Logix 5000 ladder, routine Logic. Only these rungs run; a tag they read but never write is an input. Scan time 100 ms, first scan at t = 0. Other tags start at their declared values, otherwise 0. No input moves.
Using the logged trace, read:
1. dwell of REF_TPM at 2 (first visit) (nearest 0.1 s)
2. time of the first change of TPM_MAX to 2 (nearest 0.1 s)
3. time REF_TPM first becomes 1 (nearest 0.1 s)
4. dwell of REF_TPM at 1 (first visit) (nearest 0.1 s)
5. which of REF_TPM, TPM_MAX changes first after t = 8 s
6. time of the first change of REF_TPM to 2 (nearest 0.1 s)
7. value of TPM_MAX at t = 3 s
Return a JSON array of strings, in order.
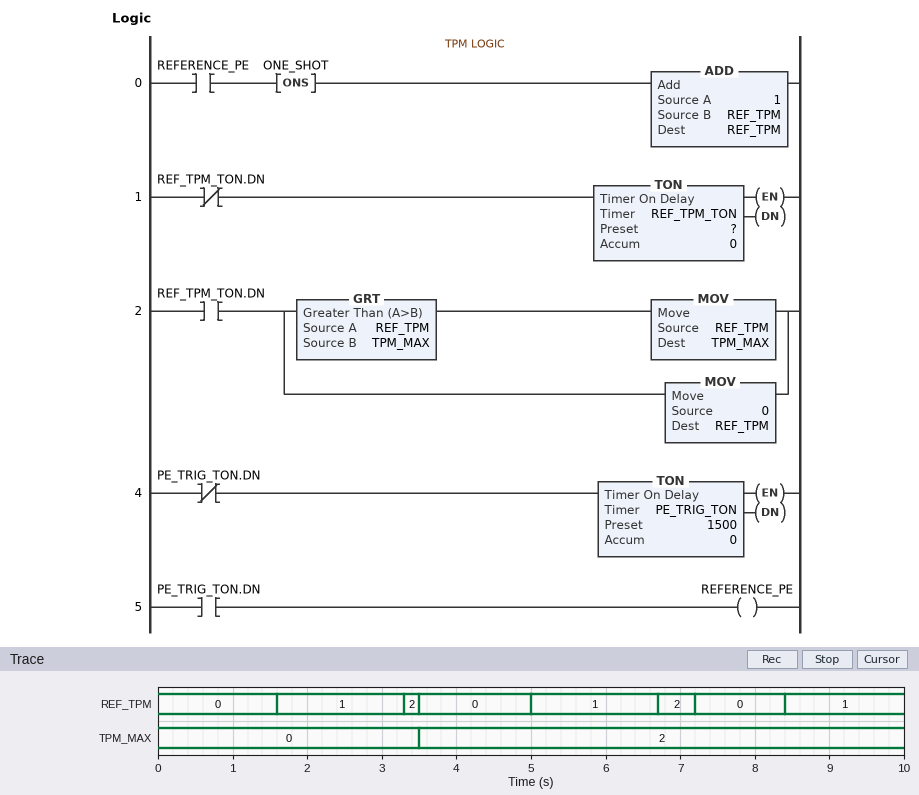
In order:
["0.2 s", "3.5 s", "1.6 s", "1.7 s", "REF_TPM", "3.3 s", "0"]
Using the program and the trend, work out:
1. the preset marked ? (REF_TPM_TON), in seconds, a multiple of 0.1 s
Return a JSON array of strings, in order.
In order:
["3.5 s"]
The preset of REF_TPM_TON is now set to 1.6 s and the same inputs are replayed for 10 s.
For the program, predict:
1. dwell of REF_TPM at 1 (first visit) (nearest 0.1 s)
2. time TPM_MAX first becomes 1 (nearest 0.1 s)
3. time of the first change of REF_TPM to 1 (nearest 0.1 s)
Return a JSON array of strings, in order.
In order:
["0.1 s", "1.6 s", "3.3 s"]
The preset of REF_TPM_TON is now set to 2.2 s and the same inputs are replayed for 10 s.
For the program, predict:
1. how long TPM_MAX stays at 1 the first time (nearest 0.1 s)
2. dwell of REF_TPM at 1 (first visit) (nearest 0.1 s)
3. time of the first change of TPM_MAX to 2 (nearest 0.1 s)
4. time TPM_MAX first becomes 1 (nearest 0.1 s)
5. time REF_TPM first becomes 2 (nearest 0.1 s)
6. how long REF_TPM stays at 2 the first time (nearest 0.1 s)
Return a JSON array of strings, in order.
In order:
["4.8 s", "0.6 s", "7.0 s", "2.2 s", "6.7 s", "0.3 s"]
